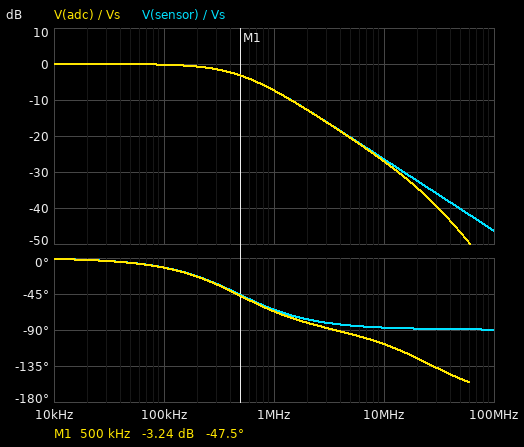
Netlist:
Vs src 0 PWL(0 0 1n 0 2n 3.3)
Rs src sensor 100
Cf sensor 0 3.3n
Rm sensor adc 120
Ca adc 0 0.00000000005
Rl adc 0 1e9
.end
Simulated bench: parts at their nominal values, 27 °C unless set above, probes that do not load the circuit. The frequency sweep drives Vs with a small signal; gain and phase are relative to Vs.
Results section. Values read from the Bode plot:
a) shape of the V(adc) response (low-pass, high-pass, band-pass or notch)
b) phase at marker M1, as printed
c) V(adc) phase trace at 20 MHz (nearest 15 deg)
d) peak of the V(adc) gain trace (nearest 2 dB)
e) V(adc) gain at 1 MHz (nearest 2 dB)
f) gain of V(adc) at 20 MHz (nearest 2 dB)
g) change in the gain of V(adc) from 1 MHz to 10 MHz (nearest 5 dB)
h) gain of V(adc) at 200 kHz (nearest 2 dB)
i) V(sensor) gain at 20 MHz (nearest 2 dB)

low-pass
-47.5 deg
-120 deg
0 dB
-8 dB
-34 dB
-20 dB
0 dB
-32 dB
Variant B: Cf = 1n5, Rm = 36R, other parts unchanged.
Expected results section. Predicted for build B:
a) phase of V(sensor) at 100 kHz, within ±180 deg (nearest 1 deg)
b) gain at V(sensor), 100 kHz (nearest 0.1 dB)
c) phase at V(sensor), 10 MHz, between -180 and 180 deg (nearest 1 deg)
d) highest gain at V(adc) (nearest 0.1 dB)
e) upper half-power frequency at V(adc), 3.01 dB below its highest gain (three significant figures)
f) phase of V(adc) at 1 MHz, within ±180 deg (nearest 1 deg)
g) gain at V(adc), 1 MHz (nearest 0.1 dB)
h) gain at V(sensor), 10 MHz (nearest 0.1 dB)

-6 deg
0 dB
-84 deg
0 dB
1.03 MHz
-45 deg
-2.9 dB
-19.8 dB
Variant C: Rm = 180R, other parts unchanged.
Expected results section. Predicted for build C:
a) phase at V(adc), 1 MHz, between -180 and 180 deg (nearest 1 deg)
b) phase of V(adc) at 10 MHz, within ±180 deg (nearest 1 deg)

-68 deg
-116 deg
